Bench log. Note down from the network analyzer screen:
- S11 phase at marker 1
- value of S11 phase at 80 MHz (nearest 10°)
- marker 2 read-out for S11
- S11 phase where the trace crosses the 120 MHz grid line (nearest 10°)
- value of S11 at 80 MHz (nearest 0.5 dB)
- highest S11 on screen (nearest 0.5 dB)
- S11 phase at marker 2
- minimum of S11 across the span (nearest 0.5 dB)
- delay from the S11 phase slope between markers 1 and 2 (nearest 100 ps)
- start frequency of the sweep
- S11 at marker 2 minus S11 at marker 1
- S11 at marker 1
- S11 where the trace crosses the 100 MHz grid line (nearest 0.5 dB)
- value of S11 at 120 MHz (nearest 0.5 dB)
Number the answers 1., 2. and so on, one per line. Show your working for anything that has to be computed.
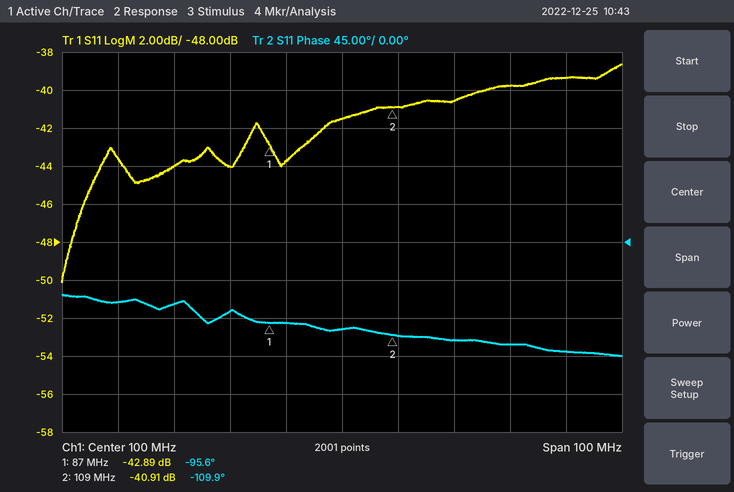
1. -95.6°
2. -80°
3. -40.91 dB
4. -120°
5. -44.0 dB
6. -38.5 dB
7. -109.9°
8. -50.0 dB
9. −(-109.9° − (-95.6°))/(360° × 22 MHz) ≈ 1.8 ns
10. 50 MHz
11. -40.91 − (-42.89) = 1.98 dB
12. -42.89 dB
13. -41.5 dB
14. -40.5 dB
